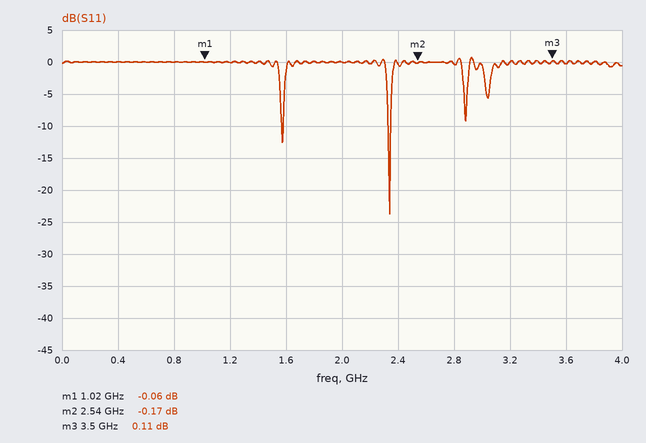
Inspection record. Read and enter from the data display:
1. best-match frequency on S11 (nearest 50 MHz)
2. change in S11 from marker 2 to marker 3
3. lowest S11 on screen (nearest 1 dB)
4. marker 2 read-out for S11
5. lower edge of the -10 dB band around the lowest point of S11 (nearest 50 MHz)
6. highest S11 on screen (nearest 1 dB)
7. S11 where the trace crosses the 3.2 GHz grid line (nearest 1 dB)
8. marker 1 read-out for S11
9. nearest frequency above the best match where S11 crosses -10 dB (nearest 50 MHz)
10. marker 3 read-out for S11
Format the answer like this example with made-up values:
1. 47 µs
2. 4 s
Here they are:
1. 2.35 GHz
2. 0.28 dB
3. -24 dB
4. -0.17 dB
5. 2.35 GHz
6. 1 dB
7. 0 dB
8. -0.06 dB
9. 2.35 GHz
10. 0.11 dB
